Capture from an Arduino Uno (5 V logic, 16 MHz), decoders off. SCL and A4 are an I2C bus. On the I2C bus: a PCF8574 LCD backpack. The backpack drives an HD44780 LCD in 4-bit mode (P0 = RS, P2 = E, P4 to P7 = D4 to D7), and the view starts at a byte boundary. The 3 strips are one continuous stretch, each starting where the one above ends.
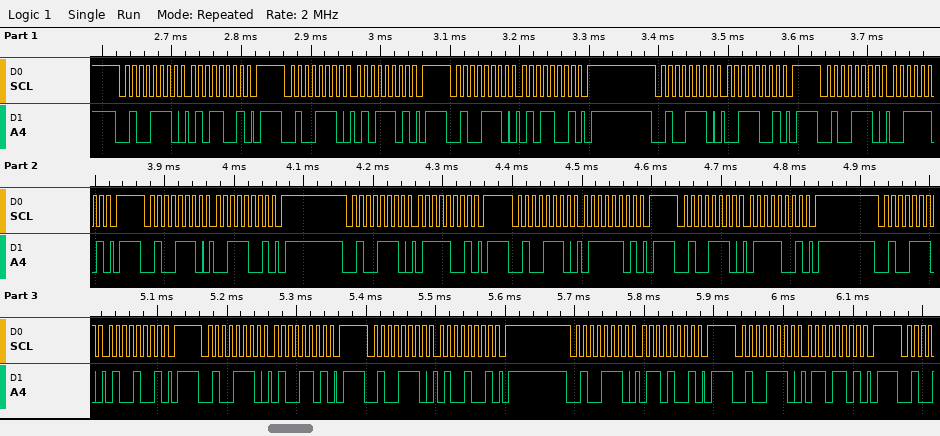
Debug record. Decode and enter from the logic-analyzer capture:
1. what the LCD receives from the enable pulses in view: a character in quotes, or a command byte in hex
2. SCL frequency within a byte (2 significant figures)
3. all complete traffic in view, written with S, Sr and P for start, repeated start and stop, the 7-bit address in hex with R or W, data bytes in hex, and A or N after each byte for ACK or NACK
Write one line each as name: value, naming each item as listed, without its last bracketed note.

what the LCD receives from the enable pulses in view: a character in quotes, or a command byte in hex: 'S' 't'
SCL frequency within a byte: 100 kHz
all complete traffic in view, written with S, Sr and P for start, repeated start and stop, the 7-bit address in hex with R or W, data bytes in hex, and A or N after each byte for ACK or NACK: S 27W A 59 A P S 27W A 5D A P S 27W A 59 A P S 27W A 39 A P S 27W A 3D A P S 27W A 39 A P S 27W A 79 A P S 27W A 7D A P S 27W A 79 A P S 27W A 49 A P S 27W A 4D A P S 27W A 49 A P S 27W A 69 A P S 27W A 6D A P
